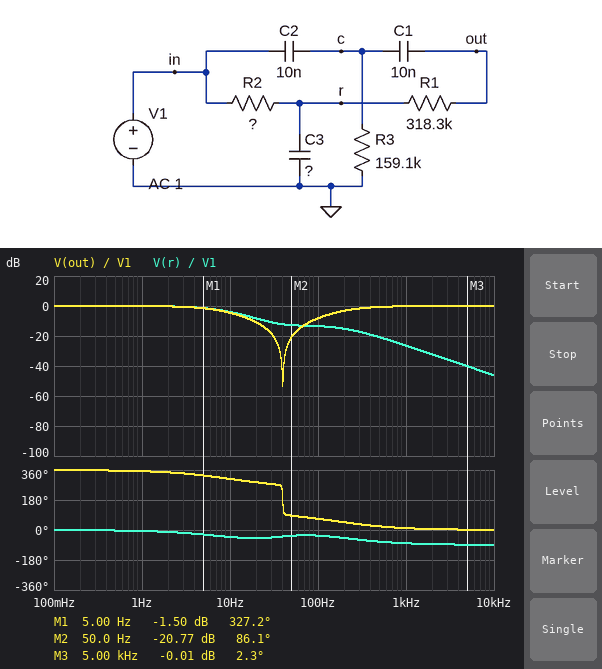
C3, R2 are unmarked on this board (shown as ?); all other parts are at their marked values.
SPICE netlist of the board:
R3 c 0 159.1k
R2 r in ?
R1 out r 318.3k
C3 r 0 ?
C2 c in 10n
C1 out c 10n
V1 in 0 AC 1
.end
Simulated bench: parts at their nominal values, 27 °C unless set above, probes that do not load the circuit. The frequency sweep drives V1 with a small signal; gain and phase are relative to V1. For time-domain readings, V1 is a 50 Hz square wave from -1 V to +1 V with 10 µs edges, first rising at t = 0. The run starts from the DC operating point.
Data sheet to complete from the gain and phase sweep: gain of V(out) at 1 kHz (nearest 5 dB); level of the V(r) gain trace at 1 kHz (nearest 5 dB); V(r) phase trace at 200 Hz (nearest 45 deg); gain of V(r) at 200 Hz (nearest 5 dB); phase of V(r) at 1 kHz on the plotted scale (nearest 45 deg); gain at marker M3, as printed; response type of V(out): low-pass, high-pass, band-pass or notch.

0 dB
-25 dB
-45 deg
-15 dB
-90 deg
-0.01 dB
notch
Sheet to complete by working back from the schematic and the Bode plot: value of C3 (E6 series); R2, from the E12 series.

15 nF
680 kΩ
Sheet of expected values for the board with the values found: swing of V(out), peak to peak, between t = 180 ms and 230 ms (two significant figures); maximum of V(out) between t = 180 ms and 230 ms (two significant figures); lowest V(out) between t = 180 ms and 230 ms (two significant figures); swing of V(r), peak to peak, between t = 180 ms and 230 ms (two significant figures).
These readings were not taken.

3.6 V
1.8 V
-1.8 V
690 mV
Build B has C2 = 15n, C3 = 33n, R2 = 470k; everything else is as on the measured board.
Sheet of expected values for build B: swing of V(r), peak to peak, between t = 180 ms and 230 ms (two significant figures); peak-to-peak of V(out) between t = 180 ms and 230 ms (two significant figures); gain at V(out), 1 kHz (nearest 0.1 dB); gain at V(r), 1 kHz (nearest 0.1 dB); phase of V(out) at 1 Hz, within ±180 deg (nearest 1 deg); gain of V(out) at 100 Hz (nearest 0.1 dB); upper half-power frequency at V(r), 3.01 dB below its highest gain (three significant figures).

580 mV
3.8 V
-0.1 dB
-32.0 dB
-8 deg
-5.5 dB
7.25 Hz
